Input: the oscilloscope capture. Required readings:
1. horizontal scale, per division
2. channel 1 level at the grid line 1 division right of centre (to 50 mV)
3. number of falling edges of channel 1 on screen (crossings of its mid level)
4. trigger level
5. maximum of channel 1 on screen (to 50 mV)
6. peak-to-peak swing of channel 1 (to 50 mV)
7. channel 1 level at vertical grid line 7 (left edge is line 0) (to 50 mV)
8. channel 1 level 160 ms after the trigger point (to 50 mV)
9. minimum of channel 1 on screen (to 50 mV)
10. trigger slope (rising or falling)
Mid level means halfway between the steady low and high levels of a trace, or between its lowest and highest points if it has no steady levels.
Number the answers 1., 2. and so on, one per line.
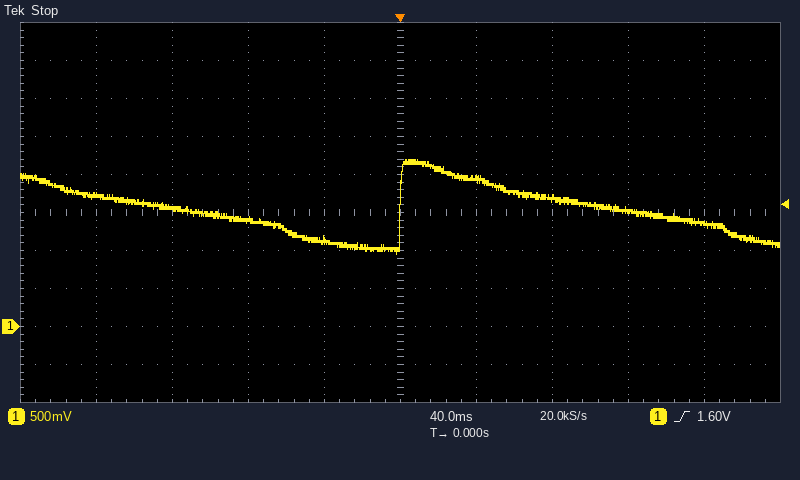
1. 40 ms
2. 1.95 V
3. 2
4. 1.60 V
5. 2.20 V
6. 1.25 V
7. 1.70 V
8. 1.35 V
9. 950 mV
10. rising
